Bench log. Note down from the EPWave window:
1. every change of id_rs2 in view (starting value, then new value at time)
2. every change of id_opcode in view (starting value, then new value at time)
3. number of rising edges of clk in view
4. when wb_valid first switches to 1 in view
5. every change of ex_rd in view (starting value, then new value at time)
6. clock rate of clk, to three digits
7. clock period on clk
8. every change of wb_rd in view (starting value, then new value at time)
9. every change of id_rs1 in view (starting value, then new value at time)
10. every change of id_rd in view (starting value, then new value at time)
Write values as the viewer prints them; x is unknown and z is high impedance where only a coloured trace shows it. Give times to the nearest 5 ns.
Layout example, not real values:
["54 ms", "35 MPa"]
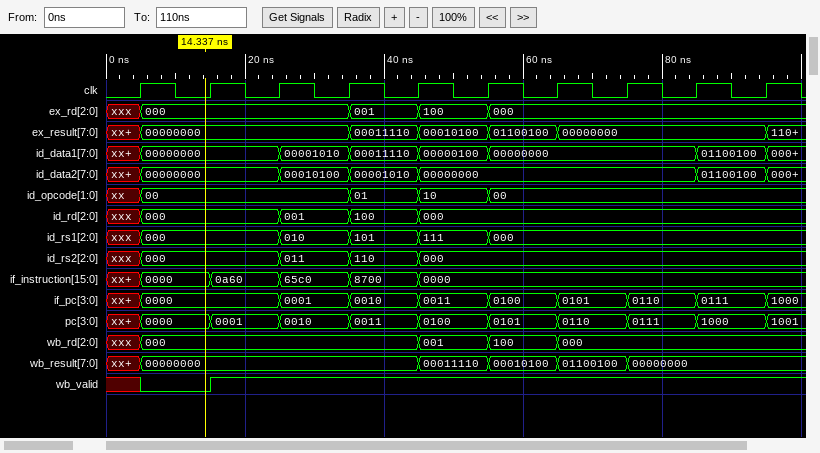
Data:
["xxx, 000 at 5 ns, 011 at 25 ns, 110 at 35 ns, 000 at 45 ns", "xx, 00 at 5 ns, 01 at 35 ns, 10 at 45 ns, 00 at 55 ns", "10", "15 ns", "xxx, 000 at 5 ns, 001 at 35 ns, 100 at 45 ns, 000 at 55 ns", "100 MHz", "10 ns", "xxx, 000 at 5 ns, 001 at 45 ns, 100 at 55 ns, 000 at 65 ns", "xxx, 000 at 5 ns, 010 at 25 ns, 101 at 35 ns, 111 at 45 ns, 000 at 55 ns", "xxx, 000 at 5 ns, 001 at 25 ns, 100 at 35 ns, 000 at 45 ns"]
